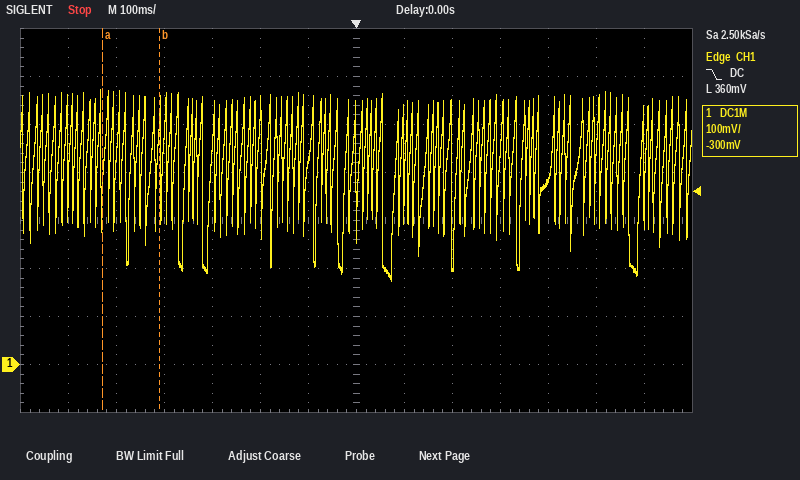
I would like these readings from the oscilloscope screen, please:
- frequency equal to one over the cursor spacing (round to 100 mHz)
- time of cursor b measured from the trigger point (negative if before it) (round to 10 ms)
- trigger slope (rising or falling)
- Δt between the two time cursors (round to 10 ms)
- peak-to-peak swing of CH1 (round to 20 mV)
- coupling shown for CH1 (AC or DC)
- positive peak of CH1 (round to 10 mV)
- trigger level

8.3 Hz
-410 ms
falling
120 ms
400 mV
DC
570 mV
360 mV
